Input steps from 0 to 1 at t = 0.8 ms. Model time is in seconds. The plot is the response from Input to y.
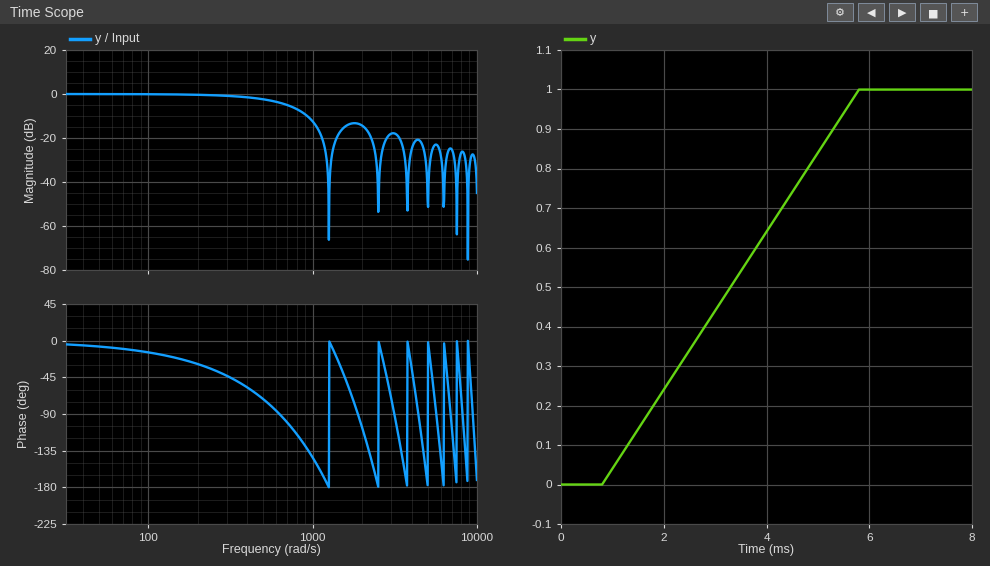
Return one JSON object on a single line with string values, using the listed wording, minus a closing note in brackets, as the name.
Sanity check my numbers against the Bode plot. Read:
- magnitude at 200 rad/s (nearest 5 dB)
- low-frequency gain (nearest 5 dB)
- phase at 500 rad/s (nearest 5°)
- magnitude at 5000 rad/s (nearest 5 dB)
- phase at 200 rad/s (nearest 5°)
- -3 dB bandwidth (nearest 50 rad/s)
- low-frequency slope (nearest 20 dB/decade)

{"magnitude at 200 rad/s": "0 dB", "low-frequency gain": "0 dB", "phase at 500 rad/s": "-70°", "magnitude at 5000 rad/s": "-45 dB", "phase at 200 rad/s": "-30°", "-3 dB bandwidth": "550 rad/s", "low-frequency slope": "0 dB/decade"}
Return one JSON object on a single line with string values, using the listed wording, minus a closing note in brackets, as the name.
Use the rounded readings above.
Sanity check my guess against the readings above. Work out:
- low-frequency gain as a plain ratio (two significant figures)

{"low-frequency gain as a plain ratio": "1.0"}
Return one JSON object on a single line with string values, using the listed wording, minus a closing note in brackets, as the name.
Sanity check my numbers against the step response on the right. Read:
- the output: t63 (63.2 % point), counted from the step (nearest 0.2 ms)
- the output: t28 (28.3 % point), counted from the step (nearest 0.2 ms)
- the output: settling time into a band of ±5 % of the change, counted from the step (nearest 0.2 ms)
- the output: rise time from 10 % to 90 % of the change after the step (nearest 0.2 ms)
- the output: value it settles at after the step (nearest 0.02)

{"the output: t63 (63.2 % point), counted from the step": "3.2 ms", "the output: t28 (28.3 % point), counted from the step": "1.4 ms", "the output: settling time into a band of ±5 % of the change, counted from the step": "4.8 ms", "the output: rise time from 10 % to 90 % of the change after the step": "4.0 ms", "the output: value it settles at after the step": "1.00"}
